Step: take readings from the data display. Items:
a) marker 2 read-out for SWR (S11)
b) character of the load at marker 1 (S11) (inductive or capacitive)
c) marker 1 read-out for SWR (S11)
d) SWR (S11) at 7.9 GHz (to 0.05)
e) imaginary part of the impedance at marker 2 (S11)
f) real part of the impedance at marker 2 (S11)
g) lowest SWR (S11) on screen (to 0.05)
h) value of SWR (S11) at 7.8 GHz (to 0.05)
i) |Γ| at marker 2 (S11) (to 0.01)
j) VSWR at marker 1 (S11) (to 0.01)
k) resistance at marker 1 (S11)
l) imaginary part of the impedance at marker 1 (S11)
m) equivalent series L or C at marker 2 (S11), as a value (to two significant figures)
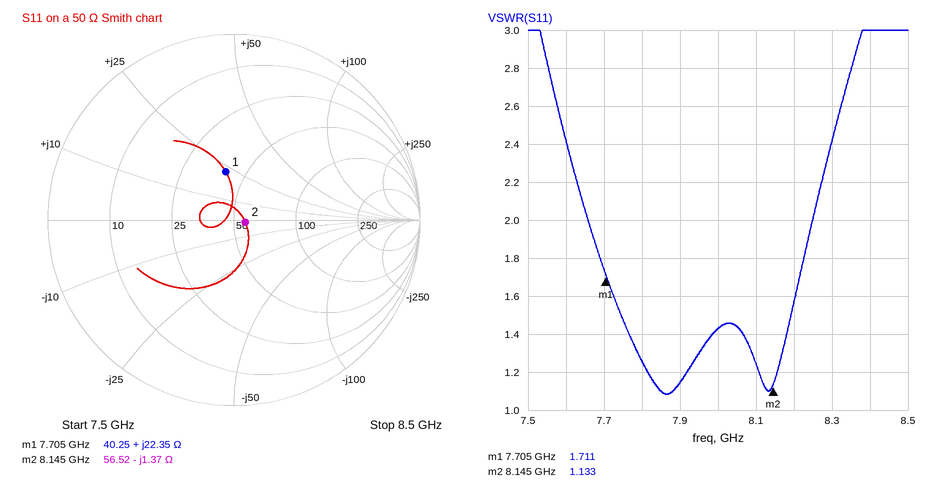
1.133
inductive
1.711
1.15
-1.37 Ω
56.52 Ω
1.10
1.25
0.06
1.71
40.25 Ω
+22.35 Ω
14 pF
